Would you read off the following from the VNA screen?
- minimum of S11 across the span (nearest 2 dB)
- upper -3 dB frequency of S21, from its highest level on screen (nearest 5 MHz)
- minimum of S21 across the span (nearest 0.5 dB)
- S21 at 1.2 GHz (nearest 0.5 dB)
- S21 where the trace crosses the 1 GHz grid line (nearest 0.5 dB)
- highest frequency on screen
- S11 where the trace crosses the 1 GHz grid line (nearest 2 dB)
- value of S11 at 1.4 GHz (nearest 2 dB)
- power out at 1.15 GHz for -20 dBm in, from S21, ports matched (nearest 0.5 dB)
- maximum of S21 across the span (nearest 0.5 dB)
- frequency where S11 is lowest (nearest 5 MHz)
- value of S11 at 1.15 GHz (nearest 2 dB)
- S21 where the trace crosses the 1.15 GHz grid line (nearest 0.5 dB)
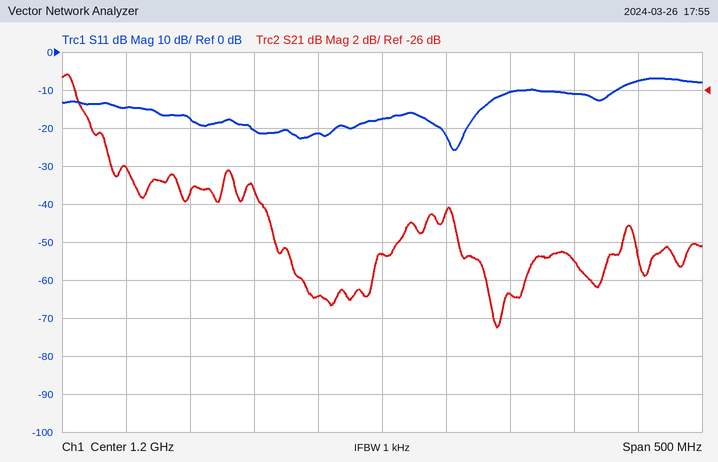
-26 dB
975 MHz
-38.5 dB
-34.5 dB
-30.0 dB
1.45 GHz
-14 dB
-8 dB
-57.0 dBm
-25.0 dB
1.255 GHz
-22 dB
-37.0 dB
